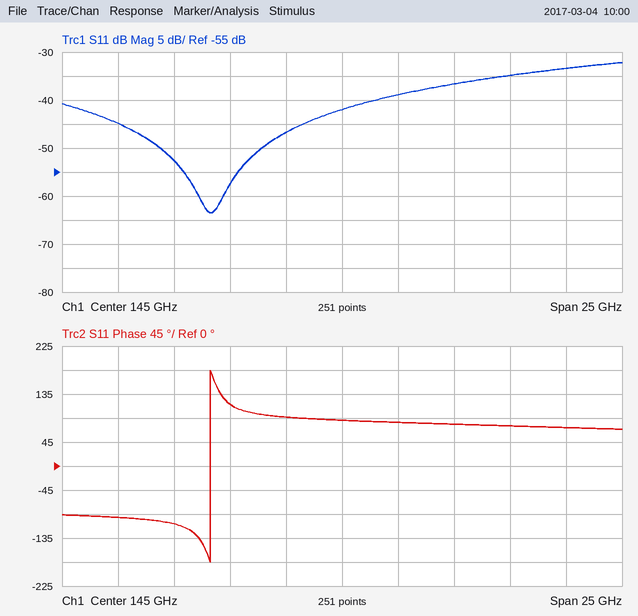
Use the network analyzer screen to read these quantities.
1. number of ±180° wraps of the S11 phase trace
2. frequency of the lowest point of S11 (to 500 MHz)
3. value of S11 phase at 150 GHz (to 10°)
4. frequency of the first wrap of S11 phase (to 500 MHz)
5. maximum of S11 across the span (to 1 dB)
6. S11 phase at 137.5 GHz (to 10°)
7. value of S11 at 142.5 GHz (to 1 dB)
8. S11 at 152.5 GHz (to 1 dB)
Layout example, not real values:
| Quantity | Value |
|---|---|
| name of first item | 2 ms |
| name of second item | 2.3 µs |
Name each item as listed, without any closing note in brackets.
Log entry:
| Quantity | Value |
|---|---|
| number of ±180° wraps of the S11 phase trace | 1 |
| frequency of the lowest point of S11 | 139.0 GHz |
| value of S11 phase at 150 GHz | 80° |
| frequency of the first wrap of S11 phase | 139.0 GHz |
| maximum of S11 across the span | -32 dB |
| S11 phase at 137.5 GHz | -110° |
| value of S11 at 142.5 GHz | -47 dB |
| S11 at 152.5 GHz | -35 dB |
